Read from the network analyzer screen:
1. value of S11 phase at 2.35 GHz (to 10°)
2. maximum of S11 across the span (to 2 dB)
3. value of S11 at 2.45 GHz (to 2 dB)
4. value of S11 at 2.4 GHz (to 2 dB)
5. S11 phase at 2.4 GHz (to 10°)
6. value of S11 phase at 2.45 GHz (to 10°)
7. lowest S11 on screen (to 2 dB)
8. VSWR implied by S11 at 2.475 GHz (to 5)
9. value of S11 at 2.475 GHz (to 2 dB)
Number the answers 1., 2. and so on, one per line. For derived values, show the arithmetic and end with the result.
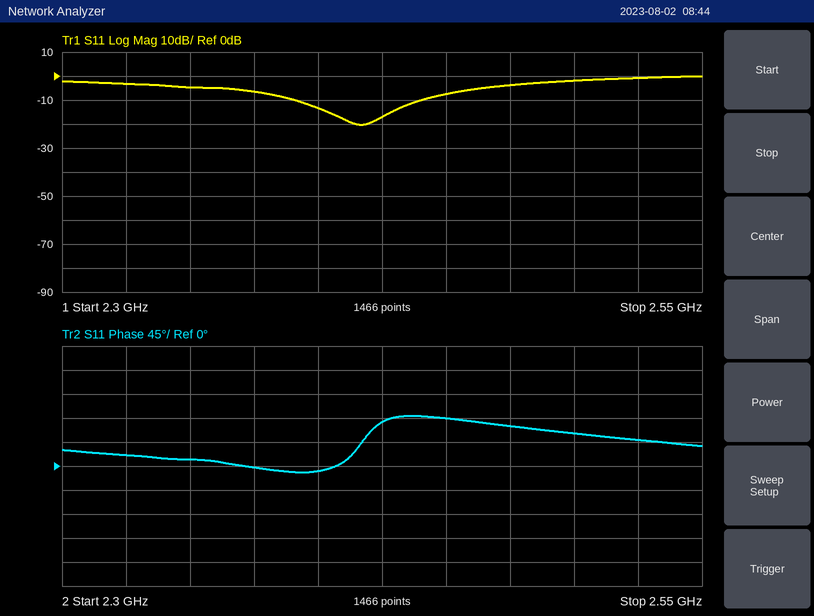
1. 10°
2. 0 dB
3. -8 dB
4. -14 dB
5. -10°
6. 90°
7. -20 dB
8. |Γ| = 10^(-4/20) = 0.6310; VSWR = (1 + 0.6310)/(1 − 0.6310) ≈ 4.42, so 5 to the nearest 5
9. -4 dB
